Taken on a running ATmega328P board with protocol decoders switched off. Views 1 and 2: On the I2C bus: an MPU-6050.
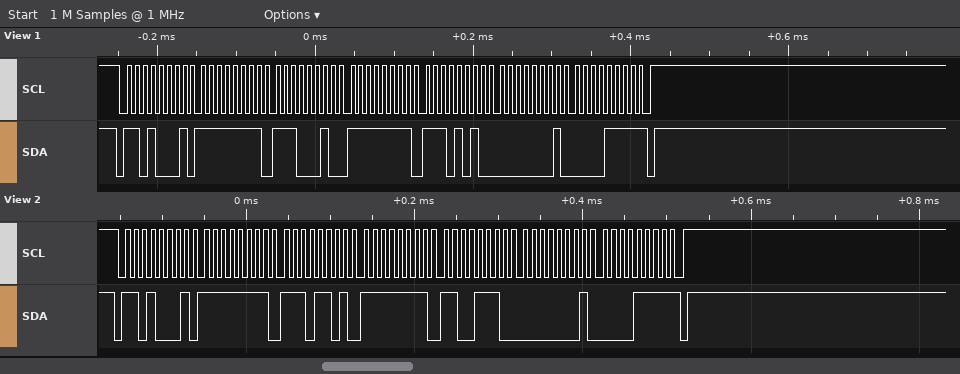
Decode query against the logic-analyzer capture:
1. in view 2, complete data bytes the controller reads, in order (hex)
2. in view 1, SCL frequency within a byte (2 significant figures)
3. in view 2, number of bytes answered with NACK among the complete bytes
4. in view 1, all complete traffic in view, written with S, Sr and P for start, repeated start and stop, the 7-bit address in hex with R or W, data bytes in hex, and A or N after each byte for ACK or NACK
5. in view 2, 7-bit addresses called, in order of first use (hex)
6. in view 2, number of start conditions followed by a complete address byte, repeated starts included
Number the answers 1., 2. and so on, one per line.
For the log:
1. FF ED FF CE 01 0F
2. 100 kHz
3. 1
4. S 68R A FF A E2 A FF A EA A 01 A 0F N P
5. 0x68
6. 1
